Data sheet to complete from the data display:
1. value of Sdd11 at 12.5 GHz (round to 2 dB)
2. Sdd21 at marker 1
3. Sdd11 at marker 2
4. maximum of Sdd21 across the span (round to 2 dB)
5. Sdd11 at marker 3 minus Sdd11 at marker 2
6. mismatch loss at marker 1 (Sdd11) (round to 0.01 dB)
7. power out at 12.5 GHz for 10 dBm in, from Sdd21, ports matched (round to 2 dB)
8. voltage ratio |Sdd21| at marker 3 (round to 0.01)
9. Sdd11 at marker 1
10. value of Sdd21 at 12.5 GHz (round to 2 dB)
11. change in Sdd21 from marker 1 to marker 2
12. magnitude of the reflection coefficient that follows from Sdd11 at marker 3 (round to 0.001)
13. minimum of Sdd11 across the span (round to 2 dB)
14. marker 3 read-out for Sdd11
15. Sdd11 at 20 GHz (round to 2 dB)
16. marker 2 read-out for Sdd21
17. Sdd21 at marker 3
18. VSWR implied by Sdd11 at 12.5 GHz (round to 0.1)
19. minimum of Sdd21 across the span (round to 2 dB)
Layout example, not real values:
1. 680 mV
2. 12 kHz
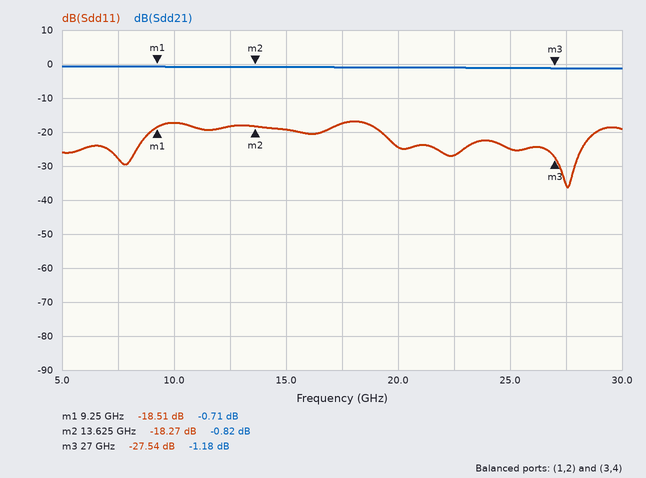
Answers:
1. -18 dB
2. -0.71 dB
3. -18.27 dB
4. 0 dB
5. -9.27 dB
6. 0.06 dB
7. 10 dBm
8. 0.87
9. -18.51 dB
10. 0 dB
11. -0.11 dB
12. 0.042
13. -36 dB
14. -27.54 dB
15. -24 dB
16. -0.82 dB
17. -1.18 dB
18. 1.3
19. -2 dB
